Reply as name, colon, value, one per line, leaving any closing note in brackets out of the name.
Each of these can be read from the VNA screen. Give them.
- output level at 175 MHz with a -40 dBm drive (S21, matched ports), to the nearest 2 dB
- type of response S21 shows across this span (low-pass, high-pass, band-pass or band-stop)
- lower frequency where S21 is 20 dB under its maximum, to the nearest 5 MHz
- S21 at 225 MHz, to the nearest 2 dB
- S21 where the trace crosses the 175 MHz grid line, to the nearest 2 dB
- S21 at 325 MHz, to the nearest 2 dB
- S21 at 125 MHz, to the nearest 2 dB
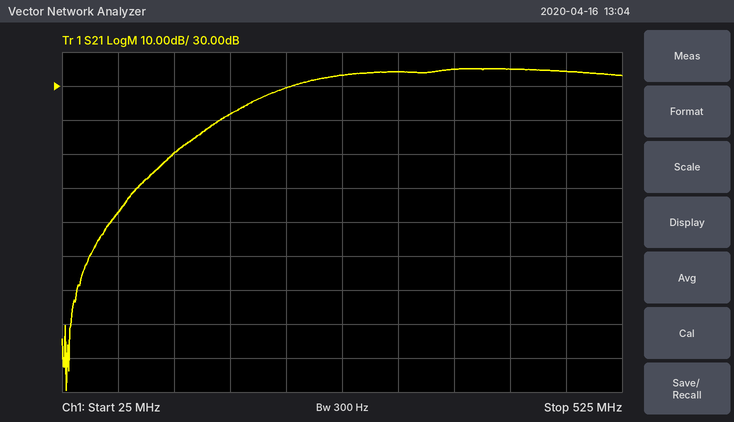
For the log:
output level at 175 MHz with a -40 dBm drive (S21, matched ports), to the nearest 2 dB: -18 dBm
type of response S21 shows across this span: high-pass
lower frequency where S21 is 20 dB under its maximum, to the nearest 5 MHz: 145 MHz
S21 at 225 MHz, to the nearest 2 dB: 30 dB
S21 where the trace crosses the 175 MHz grid line, to the nearest 2 dB: 22 dB
S21 at 325 MHz, to the nearest 2 dB: 34 dB
S21 at 125 MHz, to the nearest 2 dB: 10 dB
